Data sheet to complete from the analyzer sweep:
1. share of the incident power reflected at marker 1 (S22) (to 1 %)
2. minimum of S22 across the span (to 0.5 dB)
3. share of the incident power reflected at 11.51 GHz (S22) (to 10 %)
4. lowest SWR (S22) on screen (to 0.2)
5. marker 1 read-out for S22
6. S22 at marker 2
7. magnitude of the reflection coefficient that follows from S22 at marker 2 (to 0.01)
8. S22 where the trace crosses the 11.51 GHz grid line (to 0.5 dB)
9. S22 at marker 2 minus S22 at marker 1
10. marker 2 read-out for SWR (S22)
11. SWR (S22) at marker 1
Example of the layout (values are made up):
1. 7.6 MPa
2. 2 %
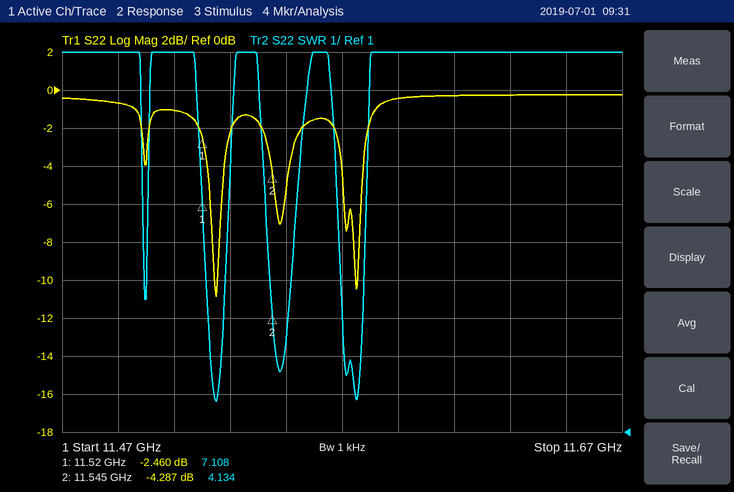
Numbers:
1. 57 %
2. -11.0 dB
3. 80 %
4. 1.8
5. -2.460 dB
6. -4.287 dB
7. 0.61
8. -1.0 dB
9. -1.827 dB
10. 4.134
11. 7.108
